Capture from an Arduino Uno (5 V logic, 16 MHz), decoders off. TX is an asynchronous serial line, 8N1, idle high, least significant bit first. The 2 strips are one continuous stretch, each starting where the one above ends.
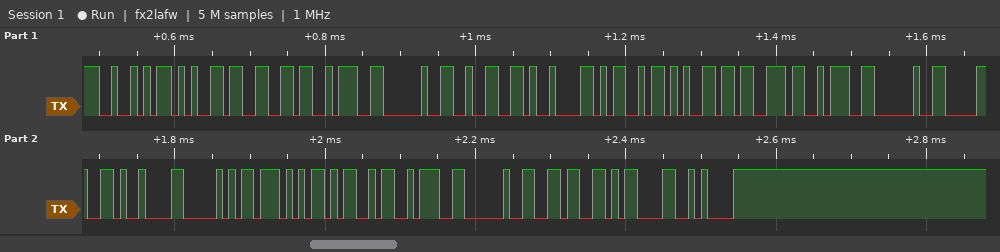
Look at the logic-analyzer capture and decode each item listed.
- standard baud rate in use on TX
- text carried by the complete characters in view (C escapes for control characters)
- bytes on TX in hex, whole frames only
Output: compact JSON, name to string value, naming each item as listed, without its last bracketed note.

{"standard baud rate in use on TX": "115200 baud", "text carried by the complete characters in view": "\"Ref: 2\\tMes: 0\\tPWM: 6\\r\\n\"", "bytes on TX in hex, whole frames only": "52 65 66 3A 20 32 09 4D 65 73 3A 20 30 09 50 57 4D 3A 20 36 0D 0A"}
